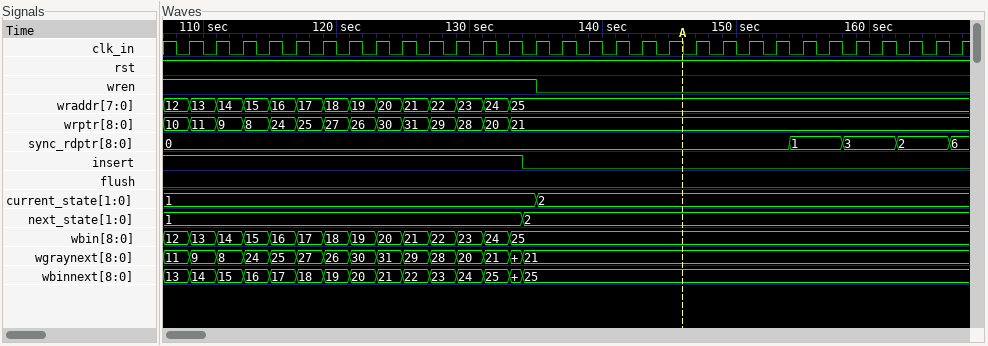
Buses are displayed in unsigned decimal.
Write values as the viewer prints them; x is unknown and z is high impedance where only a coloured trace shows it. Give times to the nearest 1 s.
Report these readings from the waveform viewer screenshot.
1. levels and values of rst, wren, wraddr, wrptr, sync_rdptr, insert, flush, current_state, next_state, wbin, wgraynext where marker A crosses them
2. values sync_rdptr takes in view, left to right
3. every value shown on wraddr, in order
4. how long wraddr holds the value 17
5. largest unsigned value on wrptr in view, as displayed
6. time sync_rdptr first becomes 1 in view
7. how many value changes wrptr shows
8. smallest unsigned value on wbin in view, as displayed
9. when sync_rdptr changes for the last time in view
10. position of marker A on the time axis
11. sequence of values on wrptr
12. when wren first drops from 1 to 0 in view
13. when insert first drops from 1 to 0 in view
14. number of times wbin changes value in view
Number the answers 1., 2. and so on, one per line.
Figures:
1. rst=1, wren=0, wraddr=25, wrptr=21, sync_rdptr=0, insert=0, flush=0, current_state=2, next_state=2, wbin=25, wgraynext=21
2. 0, 1, 3, 2, 6
3. 12, 13, 14, 15, 16, 17, 18, 19, 20, 21, 22, 23, 24, 25
4. 2 s
5. 31
6. 154 s
7. 13
8. 12
9. 166 s
10. 146 s
11. 10, 11, 9, 8, 24, 25, 27, 26, 30, 31, 29, 28, 20, 21
12. 135 s
13. 134 s
14. 13
